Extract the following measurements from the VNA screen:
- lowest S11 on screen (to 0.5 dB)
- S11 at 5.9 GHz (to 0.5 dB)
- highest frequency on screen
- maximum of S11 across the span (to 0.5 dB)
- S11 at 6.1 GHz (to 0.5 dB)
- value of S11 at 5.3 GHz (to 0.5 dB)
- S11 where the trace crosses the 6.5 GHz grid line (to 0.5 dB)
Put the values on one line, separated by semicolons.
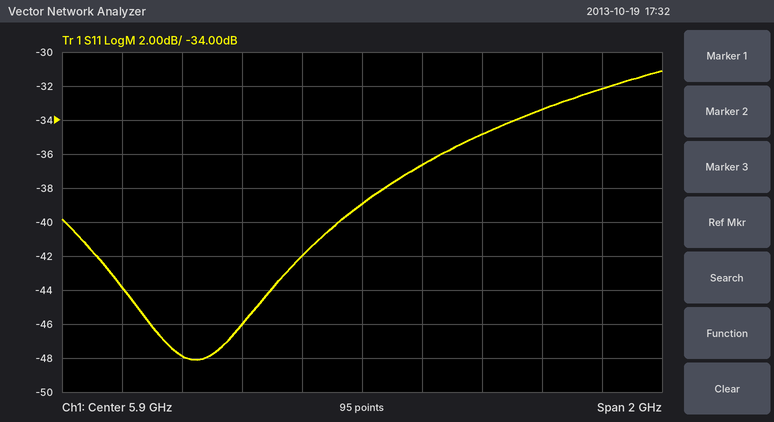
-48.0 dB; -39.0 dB; 6.9 GHz; -31.0 dB; -36.5 dB; -48.0 dB; -33.5 dB
